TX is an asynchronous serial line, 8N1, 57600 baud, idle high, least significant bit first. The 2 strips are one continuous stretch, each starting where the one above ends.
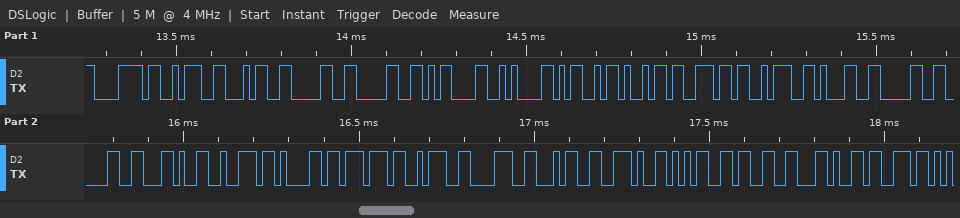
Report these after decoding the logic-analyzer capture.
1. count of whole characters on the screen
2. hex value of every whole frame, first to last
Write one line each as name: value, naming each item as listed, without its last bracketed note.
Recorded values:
count of whole characters on the screen: 26
hex value of every whole frame, first to last: 78 3A 34 30 30 0D 0A 4D 69 6E 3A 31 30 30 2C 72 61 77 3A 38 34 2E 35 33 2C 73
